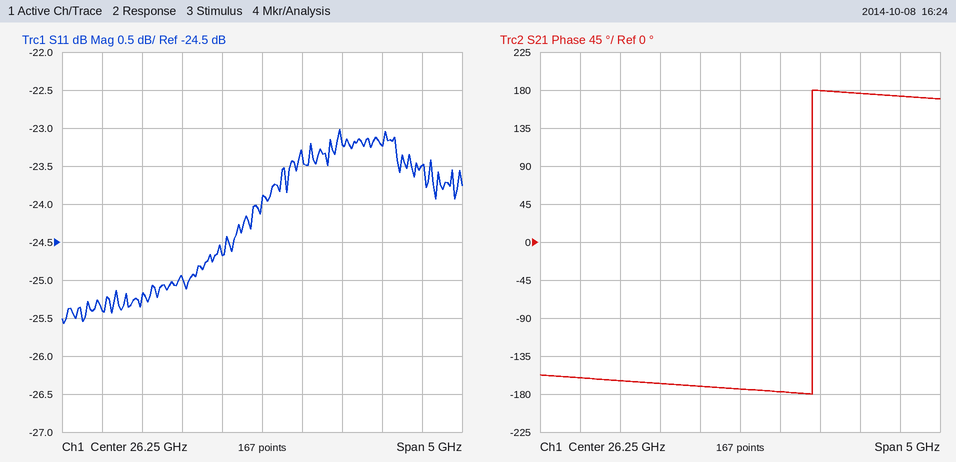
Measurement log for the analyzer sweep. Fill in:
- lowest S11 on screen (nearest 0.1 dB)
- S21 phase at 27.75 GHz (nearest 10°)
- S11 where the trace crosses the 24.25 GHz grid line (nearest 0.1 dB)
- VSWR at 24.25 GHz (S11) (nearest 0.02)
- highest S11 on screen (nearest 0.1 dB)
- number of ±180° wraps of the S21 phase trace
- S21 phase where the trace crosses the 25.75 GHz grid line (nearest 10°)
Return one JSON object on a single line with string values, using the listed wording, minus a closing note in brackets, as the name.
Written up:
{"lowest S11 on screen": "-25.6 dB", "S21 phase at 27.75 GHz": "180°", "S11 where the trace crosses the 24.25 GHz grid line": "-25.4 dB", "VSWR at 24.25 GHz (S11)": "1.12", "highest S11 on screen": "-23.0 dB", "number of ±180° wraps of the S21 phase trace": "1", "S21 phase where the trace crosses the 25.75 GHz grid line": "-170°"}
